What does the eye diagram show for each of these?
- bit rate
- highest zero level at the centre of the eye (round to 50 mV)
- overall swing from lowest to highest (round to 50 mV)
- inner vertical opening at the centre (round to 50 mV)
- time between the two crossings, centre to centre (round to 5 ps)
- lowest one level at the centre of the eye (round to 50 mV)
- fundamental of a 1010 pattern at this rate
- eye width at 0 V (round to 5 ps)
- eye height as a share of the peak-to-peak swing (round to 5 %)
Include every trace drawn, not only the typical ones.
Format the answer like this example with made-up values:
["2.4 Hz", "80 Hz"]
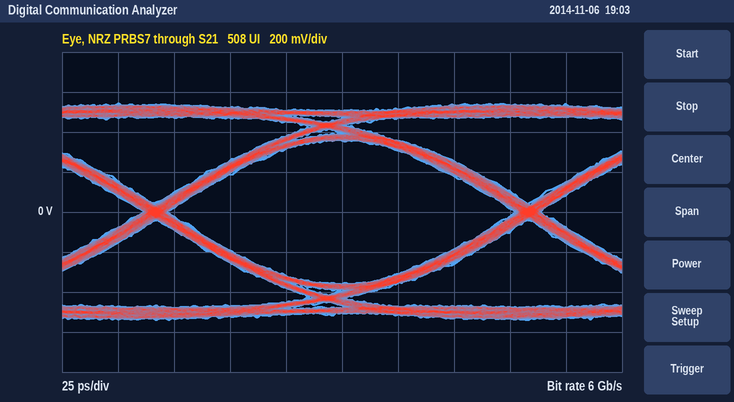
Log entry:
["6 Gb/s", "-350 mV", "1.10 V", "700 mV", "165 ps", "350 mV", "3 GHz", "155 ps", "65 %"]
